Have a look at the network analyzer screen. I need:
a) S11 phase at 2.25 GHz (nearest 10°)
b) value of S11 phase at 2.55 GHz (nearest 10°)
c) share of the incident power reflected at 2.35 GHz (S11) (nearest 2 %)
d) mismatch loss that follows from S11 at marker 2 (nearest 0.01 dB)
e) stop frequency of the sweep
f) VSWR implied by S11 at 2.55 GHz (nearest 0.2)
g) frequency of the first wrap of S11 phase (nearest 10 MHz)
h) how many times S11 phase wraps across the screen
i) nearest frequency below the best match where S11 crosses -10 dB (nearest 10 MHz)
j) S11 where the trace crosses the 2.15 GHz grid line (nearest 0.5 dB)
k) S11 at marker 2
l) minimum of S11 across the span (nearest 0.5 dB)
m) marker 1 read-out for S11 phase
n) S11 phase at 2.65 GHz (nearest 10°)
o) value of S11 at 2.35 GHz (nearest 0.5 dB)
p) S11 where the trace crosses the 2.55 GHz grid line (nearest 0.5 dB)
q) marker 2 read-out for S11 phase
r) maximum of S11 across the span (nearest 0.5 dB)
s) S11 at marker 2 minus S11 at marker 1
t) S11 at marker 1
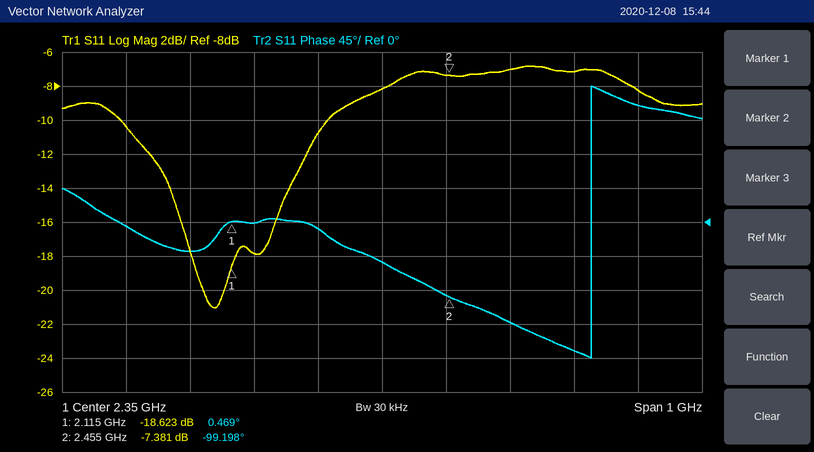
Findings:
-10°
-130°
16 %
0.88 dB
2.85 GHz
2.6
2.68 GHz
1
1.94 GHz
-18.0 dB
-7.381 dB
-21.0 dB
0.469°
-170°
-8.0 dB
-7.0 dB
-99.198°
-7.0 dB
11.242 dB
-18.623 dB
